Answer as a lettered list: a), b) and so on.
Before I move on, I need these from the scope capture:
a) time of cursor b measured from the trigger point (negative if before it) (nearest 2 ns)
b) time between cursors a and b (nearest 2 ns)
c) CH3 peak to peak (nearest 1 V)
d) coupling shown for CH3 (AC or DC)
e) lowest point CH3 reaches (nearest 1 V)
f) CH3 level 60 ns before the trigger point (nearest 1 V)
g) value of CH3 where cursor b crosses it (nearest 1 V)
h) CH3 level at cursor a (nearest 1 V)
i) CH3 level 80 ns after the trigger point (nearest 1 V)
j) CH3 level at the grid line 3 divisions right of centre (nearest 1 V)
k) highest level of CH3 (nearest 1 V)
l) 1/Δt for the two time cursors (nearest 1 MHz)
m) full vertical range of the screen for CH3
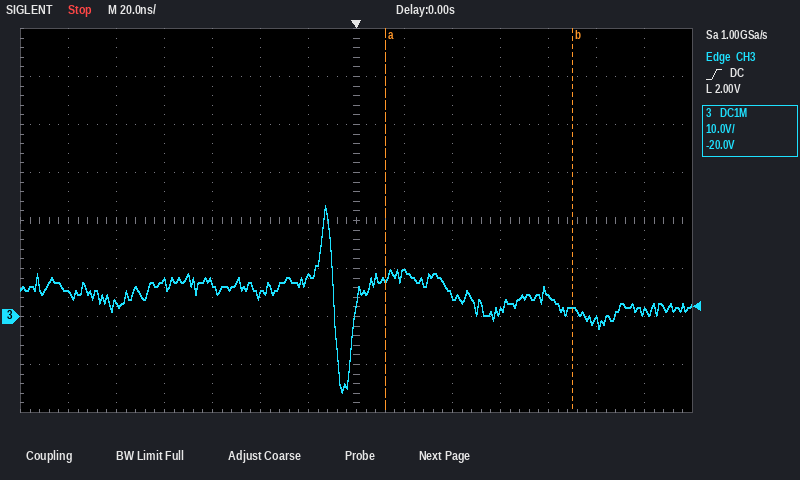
a) +90 ns
b) 78 ns
c) 39 V
d) DC
e) -16 V
f) 7 V
g) 2 V
h) 8 V
i) 4 V
j) 1 V
k) 23 V
l) 13 MHz
m) 80 V
